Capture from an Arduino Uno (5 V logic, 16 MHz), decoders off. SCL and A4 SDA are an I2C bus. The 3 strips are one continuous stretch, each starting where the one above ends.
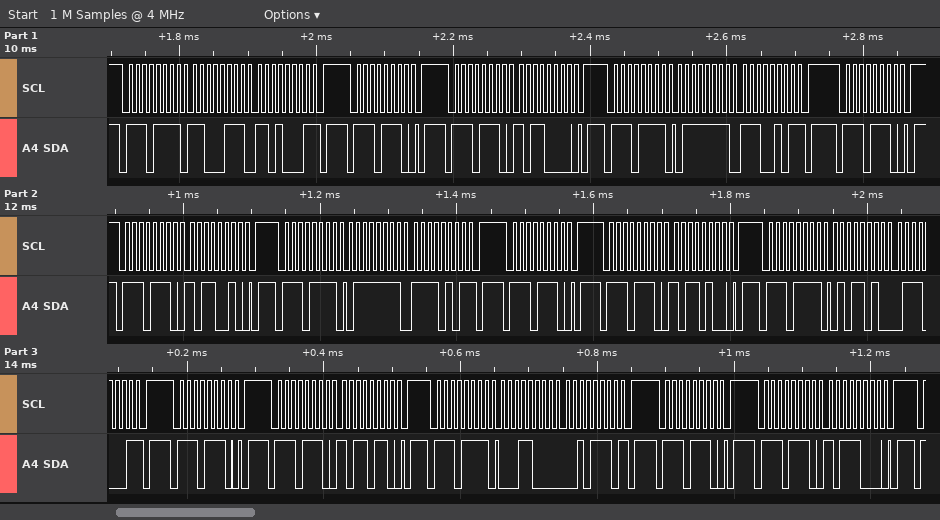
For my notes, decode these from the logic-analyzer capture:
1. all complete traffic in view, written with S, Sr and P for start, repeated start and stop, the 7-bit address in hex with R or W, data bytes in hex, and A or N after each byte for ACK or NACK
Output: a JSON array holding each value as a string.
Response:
["S 77R A C7 A D1 N P S 77W A P S 77W A B0 A P S 77R A 7F A E5 N P S 77W A P S 77W A B2 A P S 77R A 7F A F5 N P S 77W A P S 77W A B4 A P S 77R A 5A A 71 N P S 77W A P S 77W A B6 A P S 77R A 18 A 2E N P S 77W A P S 77W A B8 A P"]
